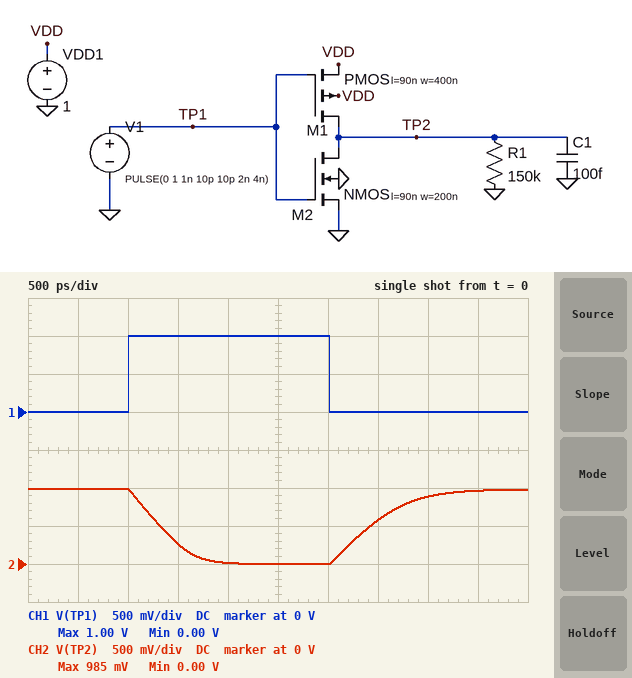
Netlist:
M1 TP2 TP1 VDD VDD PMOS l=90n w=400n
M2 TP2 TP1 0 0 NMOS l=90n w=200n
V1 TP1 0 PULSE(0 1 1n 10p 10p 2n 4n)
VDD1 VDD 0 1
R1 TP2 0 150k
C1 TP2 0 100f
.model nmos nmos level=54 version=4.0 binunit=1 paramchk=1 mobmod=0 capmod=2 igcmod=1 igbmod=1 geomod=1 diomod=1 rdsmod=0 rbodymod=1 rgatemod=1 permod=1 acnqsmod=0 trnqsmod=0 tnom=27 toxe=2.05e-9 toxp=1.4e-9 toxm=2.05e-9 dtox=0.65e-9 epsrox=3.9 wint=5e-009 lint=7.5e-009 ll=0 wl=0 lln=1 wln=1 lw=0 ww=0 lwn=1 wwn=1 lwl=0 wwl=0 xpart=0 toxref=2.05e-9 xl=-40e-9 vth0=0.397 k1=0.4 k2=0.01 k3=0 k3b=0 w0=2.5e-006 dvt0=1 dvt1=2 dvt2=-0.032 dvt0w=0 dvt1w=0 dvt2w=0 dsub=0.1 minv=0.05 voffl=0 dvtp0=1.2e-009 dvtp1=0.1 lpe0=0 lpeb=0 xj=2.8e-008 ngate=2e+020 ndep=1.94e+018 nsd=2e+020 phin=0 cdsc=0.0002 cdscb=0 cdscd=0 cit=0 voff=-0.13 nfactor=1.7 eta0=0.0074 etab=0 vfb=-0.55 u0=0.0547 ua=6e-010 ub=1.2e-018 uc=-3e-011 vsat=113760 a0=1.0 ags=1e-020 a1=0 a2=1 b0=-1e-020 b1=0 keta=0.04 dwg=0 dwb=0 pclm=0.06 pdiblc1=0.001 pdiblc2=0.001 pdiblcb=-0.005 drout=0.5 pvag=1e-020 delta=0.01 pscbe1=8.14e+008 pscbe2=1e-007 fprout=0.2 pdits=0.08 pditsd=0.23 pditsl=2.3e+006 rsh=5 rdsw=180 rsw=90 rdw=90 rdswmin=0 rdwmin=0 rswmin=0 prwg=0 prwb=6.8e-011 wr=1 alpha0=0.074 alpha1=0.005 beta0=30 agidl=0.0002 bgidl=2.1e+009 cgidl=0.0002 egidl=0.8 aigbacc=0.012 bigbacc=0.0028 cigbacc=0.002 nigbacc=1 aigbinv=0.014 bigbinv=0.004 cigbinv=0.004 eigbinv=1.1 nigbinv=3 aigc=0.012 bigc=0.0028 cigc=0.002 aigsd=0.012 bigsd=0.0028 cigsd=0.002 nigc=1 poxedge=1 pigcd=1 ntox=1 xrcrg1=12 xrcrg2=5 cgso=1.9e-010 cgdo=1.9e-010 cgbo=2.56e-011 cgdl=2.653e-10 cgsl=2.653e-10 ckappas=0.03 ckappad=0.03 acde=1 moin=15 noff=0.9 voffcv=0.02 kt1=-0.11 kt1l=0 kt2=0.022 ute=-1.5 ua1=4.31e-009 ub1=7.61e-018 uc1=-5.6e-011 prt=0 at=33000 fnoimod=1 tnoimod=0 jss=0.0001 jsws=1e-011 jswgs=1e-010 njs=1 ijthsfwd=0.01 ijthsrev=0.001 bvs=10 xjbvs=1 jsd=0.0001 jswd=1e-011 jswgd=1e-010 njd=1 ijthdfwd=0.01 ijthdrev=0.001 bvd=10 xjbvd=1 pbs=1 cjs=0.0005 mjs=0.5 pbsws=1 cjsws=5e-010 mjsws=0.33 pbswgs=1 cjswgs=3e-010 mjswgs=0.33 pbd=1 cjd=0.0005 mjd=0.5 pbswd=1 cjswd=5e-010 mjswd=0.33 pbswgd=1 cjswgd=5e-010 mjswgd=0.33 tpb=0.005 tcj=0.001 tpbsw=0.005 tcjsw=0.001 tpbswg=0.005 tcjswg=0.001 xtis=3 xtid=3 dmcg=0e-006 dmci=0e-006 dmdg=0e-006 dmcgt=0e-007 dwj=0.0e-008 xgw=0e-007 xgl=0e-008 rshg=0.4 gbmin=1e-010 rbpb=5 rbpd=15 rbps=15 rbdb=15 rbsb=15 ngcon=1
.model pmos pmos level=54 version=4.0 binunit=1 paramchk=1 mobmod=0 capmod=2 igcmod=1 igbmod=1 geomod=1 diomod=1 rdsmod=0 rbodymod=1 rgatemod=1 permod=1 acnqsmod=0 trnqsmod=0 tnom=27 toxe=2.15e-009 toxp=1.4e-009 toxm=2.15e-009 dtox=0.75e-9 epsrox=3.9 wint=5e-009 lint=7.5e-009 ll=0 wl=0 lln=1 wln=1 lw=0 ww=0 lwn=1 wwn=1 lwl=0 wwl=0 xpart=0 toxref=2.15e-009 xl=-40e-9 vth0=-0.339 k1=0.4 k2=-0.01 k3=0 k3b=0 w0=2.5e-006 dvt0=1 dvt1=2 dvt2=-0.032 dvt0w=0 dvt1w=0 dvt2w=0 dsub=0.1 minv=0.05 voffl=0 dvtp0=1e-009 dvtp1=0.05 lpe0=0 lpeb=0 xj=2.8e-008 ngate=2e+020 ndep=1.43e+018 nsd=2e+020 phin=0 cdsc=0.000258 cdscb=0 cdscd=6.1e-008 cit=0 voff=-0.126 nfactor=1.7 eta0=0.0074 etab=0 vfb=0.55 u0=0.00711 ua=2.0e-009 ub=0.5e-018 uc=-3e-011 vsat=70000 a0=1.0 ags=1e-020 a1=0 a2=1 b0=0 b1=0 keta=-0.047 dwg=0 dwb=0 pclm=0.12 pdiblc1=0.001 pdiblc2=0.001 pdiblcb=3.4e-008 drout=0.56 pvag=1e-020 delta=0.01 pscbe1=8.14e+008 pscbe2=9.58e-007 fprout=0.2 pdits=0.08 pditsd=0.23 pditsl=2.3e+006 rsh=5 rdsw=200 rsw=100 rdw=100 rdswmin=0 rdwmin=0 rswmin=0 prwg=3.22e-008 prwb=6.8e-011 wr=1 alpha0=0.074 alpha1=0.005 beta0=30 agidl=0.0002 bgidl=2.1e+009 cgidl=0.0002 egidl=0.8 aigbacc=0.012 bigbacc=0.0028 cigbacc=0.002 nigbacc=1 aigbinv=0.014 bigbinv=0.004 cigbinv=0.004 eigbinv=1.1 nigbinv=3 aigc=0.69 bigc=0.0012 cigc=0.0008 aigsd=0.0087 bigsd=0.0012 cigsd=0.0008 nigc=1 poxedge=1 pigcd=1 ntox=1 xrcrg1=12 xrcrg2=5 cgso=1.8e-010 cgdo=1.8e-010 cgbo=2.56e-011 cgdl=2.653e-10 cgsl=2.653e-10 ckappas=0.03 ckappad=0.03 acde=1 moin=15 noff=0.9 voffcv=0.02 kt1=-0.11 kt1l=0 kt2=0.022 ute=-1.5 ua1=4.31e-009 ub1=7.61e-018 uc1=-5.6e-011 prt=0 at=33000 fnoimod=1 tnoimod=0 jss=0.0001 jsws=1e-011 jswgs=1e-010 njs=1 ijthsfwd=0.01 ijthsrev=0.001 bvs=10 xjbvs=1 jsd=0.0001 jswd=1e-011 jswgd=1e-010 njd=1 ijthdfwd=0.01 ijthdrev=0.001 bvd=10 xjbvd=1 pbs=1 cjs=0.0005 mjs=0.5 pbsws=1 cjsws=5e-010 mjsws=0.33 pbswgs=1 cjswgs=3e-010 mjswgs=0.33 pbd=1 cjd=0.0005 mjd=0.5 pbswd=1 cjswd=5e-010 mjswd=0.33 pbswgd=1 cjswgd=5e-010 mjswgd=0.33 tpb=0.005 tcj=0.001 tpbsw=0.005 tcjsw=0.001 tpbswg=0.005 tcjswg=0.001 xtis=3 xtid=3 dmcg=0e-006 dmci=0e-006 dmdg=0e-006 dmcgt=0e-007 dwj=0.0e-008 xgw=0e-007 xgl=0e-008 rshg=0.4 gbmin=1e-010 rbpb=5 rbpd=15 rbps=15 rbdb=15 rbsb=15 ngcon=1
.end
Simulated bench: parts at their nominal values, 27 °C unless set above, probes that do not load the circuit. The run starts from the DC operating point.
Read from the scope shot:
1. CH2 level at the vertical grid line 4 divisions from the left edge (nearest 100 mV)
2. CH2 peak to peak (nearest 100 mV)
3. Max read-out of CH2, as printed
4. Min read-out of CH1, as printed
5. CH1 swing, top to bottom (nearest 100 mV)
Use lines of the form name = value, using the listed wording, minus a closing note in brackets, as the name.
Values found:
CH2 level at the vertical grid line 4 divisions from the left edge = 0 V
CH2 peak to peak = 1.0 V
Max read-out of CH2, as printed = 985 mV
Min read-out of CH1, as printed = 0.00 V
CH1 swing, top to bottom = 1.0 V
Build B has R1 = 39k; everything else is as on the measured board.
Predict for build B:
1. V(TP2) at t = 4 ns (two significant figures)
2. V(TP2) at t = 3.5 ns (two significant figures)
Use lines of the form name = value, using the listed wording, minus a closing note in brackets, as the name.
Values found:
V(TP2) at t = 4 ns = 840 mV
V(TP2) at t = 3.5 ns = 550 mV
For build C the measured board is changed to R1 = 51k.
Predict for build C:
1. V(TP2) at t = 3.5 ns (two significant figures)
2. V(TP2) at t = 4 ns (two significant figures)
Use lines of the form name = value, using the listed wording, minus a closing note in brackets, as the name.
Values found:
V(TP2) at t = 3.5 ns = 560 mV
V(TP2) at t = 4 ns = 850 mV
